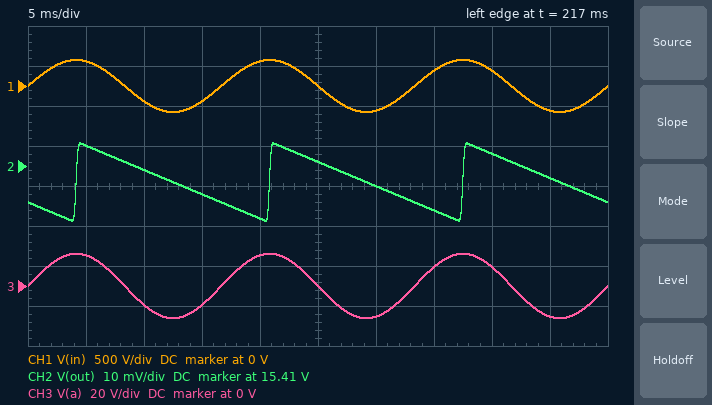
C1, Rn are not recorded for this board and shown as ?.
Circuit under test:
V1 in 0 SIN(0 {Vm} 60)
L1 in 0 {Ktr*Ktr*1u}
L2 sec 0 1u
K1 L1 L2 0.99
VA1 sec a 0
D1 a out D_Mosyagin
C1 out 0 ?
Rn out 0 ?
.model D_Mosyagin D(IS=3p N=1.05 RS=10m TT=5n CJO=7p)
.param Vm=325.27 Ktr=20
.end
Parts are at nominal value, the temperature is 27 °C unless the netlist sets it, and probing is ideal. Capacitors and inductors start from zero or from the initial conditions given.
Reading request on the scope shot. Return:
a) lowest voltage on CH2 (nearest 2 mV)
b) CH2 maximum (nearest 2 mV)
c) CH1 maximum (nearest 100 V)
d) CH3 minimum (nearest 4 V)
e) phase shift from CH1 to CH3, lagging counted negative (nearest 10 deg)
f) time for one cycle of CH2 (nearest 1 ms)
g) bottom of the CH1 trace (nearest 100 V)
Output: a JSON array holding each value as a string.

["15.396 V", "15.416 V", "300 V", "-16 V", "0 deg", "17 ms", "-300 V"]
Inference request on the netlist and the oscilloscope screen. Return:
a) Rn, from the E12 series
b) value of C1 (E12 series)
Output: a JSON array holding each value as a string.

["2.7 kΩ", "4.7 mF"]
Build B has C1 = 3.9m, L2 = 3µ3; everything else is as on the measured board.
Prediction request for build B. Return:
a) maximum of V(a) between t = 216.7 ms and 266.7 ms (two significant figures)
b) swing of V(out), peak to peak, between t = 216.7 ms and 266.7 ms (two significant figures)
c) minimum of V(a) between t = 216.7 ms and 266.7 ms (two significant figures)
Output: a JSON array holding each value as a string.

["29 V", "44 mV", "-29 V"]
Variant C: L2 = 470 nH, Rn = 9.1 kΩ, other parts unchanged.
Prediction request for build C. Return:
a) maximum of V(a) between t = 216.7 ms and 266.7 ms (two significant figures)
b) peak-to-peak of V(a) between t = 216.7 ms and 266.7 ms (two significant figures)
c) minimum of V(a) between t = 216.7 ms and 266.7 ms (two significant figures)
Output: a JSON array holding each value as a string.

["11 V", "22 V", "-11 V"]
